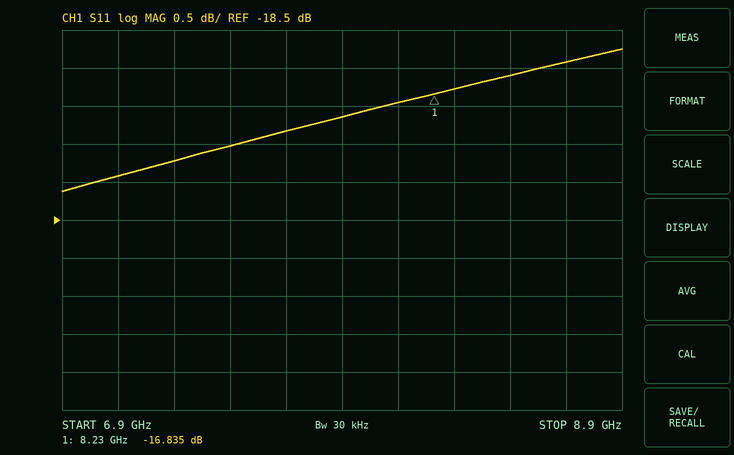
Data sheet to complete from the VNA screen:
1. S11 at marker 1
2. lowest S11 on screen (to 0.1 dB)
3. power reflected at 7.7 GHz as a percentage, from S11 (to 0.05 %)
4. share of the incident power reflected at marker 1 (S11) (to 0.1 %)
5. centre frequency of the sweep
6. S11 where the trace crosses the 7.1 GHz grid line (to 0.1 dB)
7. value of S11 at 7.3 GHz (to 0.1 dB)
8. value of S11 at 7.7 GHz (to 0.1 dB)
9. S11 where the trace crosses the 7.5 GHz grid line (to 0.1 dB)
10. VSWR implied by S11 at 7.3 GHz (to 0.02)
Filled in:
-16.835 dB
-18.1 dB
1.85 %
2.1 %
7.9 GHz
-17.9 dB
-17.7 dB
-17.3 dB
-17.5 dB
1.30
